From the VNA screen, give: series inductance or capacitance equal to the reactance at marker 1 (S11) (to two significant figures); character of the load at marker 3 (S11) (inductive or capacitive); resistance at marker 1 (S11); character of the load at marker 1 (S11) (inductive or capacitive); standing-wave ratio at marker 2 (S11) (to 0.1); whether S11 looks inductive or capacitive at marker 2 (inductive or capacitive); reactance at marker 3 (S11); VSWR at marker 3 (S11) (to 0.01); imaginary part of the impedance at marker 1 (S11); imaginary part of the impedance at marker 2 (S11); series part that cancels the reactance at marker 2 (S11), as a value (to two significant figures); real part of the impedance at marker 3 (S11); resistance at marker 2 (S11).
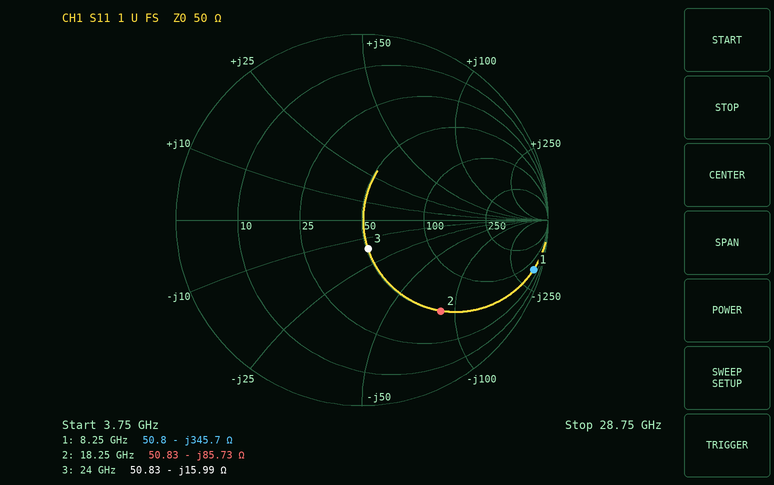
56 fF
capacitive
50.8 Ω
capacitive
4.7
capacitive
-15.99 Ω
1.37
-345.7 Ω
-85.73 Ω
750 pH
50.83 Ω
50.83 Ω
